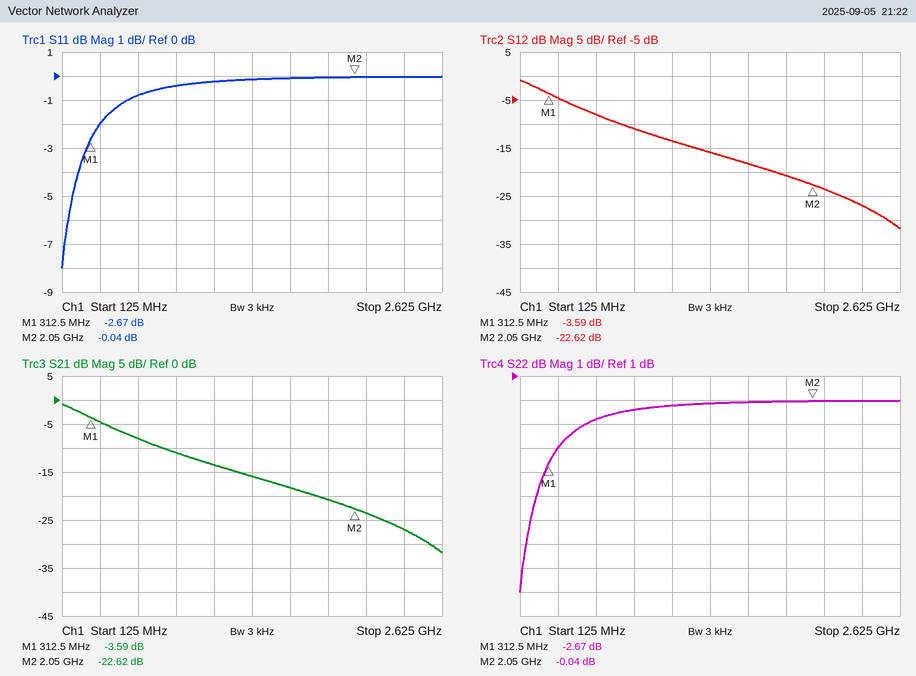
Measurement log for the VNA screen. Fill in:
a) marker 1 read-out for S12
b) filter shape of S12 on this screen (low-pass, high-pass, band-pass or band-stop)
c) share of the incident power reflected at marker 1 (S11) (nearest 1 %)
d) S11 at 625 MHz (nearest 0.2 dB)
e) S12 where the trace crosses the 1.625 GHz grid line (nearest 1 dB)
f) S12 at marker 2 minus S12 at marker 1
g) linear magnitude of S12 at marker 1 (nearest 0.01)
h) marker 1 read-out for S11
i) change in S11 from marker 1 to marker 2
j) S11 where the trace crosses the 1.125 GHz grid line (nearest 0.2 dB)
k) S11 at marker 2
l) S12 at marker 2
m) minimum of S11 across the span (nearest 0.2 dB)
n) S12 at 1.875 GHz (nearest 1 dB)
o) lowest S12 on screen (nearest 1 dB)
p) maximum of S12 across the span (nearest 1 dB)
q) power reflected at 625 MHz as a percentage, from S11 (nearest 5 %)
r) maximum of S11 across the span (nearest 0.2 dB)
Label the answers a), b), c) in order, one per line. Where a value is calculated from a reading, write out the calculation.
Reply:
a) -3.59 dB
b) low-pass
c) 10^(-2.67/10) ≈ 54 %
d) -0.8 dB
e) -18 dB
f) -22.62 − (-3.59) = -19.03 dB
g) 10^(-3.59/20) ≈ 0.66
h) -2.67 dB
i) -0.04 − (-2.67) = 2.63 dB
j) -0.2 dB
k) -0.04 dB
l) -22.62 dB
m) -8.0 dB
n) -21 dB
o) -32 dB
p) -1 dB
q) 10^(-0.8/10) ≈ 83.2 %, so 85 % to the nearest 5 %
r) 0.0 dB
